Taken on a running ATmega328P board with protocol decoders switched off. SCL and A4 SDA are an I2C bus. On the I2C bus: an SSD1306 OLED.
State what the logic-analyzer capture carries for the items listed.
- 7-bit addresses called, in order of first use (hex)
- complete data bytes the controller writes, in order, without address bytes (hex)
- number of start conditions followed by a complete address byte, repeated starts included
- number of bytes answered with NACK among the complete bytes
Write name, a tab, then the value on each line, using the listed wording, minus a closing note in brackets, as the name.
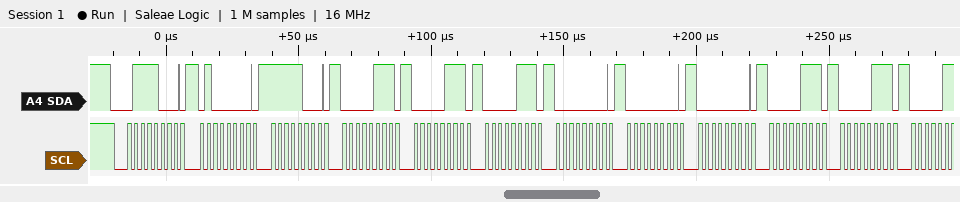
7-bit addresses called, in order of first use	0x3C
complete data bytes the controller writes, in order, without address bytes	40 F8 07 07 07 00 00 00 07 07
number of start conditions followed by a complete address byte, repeated starts included	1
number of bytes answered with NACK among the complete bytes	0
